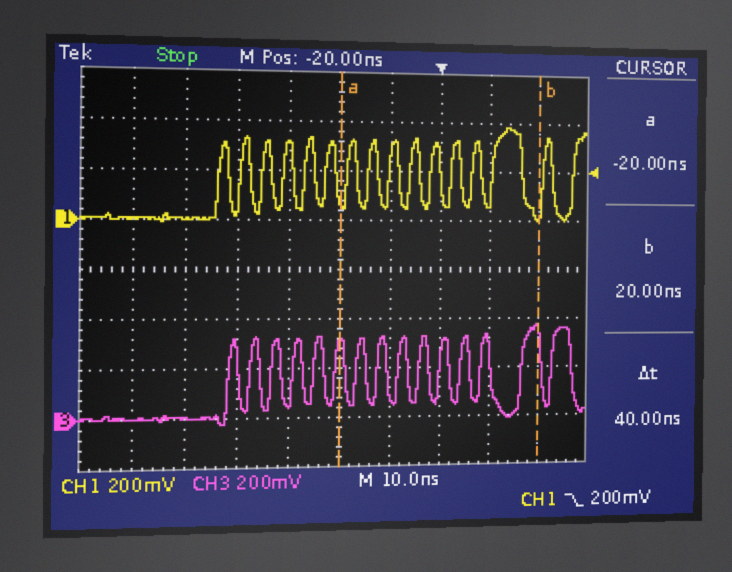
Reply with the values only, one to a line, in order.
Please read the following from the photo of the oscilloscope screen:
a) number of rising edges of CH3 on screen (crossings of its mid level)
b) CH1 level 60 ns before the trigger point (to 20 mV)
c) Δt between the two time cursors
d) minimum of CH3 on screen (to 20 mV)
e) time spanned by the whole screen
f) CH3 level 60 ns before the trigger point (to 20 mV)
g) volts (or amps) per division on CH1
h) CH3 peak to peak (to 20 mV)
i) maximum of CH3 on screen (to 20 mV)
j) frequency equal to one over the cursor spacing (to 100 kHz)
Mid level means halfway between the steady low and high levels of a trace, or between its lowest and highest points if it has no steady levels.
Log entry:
15
0 mV
40 ns
-20 mV
100 ns
0 mV
200 mV
400 mV
380 mV
25.0 MHz
